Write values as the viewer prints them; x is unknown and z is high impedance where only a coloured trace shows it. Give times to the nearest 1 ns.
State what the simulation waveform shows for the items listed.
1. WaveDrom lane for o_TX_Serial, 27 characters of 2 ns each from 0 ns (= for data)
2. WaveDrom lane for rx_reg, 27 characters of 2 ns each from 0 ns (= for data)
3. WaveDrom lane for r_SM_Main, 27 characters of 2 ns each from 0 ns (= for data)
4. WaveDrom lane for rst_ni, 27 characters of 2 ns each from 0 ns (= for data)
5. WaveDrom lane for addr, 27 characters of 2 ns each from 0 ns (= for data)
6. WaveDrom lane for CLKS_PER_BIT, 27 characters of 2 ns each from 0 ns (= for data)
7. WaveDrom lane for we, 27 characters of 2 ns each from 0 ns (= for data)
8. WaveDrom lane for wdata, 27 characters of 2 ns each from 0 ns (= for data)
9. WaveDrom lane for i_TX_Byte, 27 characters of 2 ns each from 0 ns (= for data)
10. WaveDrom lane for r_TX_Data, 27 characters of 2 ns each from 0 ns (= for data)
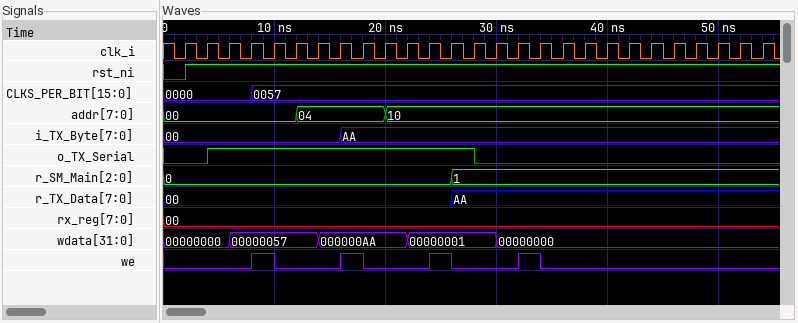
{name: 'o_TX_Serial', wave: '0.1...........0............'}
{name: 'rx_reg', wave: '=..........................', data: '00'}
{name: 'r_SM_Main', wave: '=............=.............', data: '0 1'}
{name: 'rst_ni', wave: '01.........................'}
{name: 'addr', wave: '=.....=...=................', data: '00 04 10'}
{name: 'CLKS_PER_BIT', wave: '=...=......................', data: '0000 0057'}
{name: 'we', wave: '0...10..10..10..10.........'}
{name: 'wdata', wave: '=..=...=...=...=...........', data: '00000000 00000057 000000AA 00000001 00000000'}
{name: 'i_TX_Byte', wave: '=.......=..................', data: '00 AA'}
{name: 'r_TX_Data', wave: '=............=.............', data: '00 AA'}
